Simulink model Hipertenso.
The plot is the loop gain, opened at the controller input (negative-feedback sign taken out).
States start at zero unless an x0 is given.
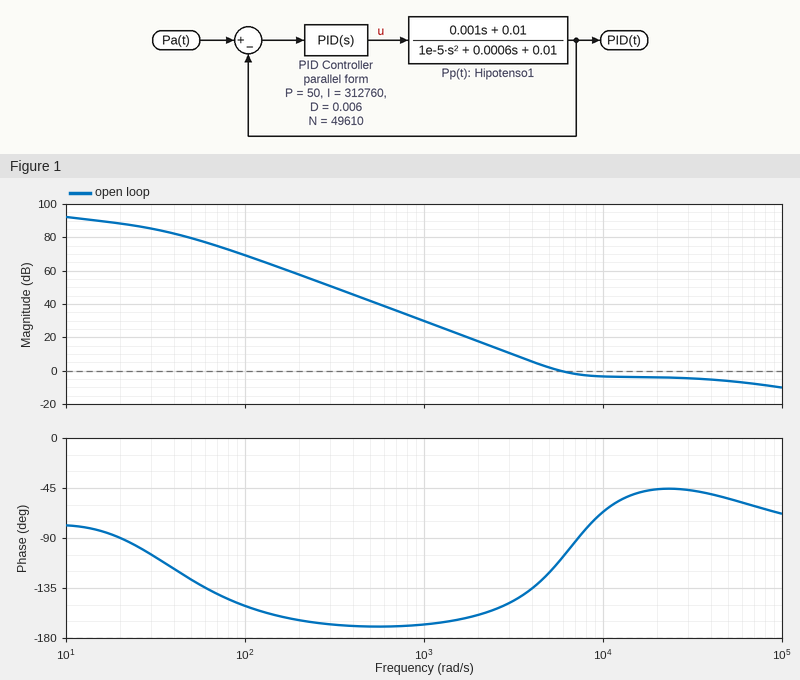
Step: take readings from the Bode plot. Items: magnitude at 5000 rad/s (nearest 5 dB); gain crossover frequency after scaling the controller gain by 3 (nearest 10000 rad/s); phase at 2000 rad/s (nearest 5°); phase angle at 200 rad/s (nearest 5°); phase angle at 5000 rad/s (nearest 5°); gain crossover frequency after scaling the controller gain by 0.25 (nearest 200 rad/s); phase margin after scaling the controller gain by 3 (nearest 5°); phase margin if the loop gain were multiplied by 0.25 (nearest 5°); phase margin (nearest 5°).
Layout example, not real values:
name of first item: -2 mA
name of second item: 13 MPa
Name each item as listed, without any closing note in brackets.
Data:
magnitude at 5000 rad/s: 0 dB
gain crossover frequency after scaling the controller gain by 3: 90000 rad/s
phase at 2000 rad/s: -160°
phase angle at 200 rad/s: -165°
phase angle at 5000 rad/s: -120°
gain crossover frequency after scaling the controller gain by 0.25: 2800 rad/s
phase margin after scaling the controller gain by 3: 115°
phase margin if the loop gain were multiplied by 0.25: 30°
phase margin: 70°
